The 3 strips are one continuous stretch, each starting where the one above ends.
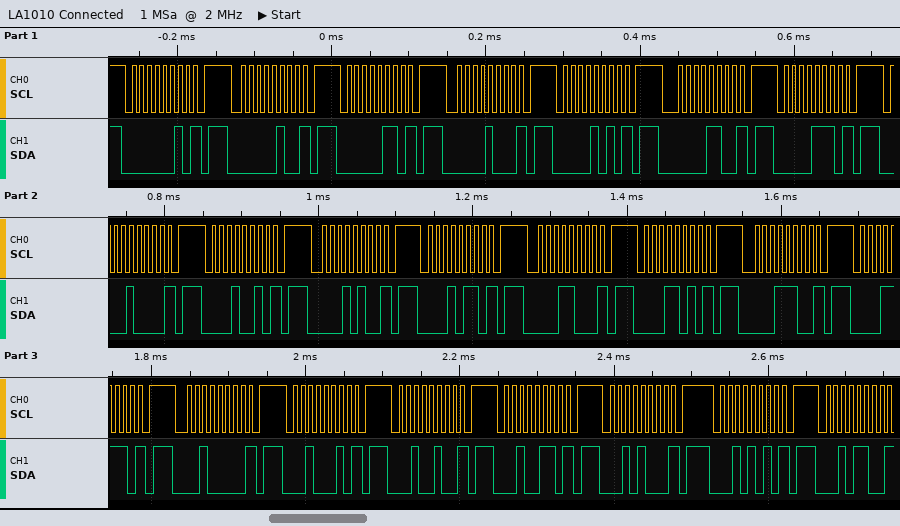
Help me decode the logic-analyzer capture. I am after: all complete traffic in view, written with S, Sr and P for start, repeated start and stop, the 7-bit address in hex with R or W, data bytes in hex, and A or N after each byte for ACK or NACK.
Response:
S 01W N P S 02W N P S 03W N P S 04W N P S 05W N P S 06W N P S 07W N P S 08W N P S 09W N P S 0AW N P S 0BW N P S 0CW N P S 0DW N P S 0EW N P S 0FW N P S 10W N P S 11W N P S 12W N P S 13W N P S 14W N P S 15W N P S 16W N
